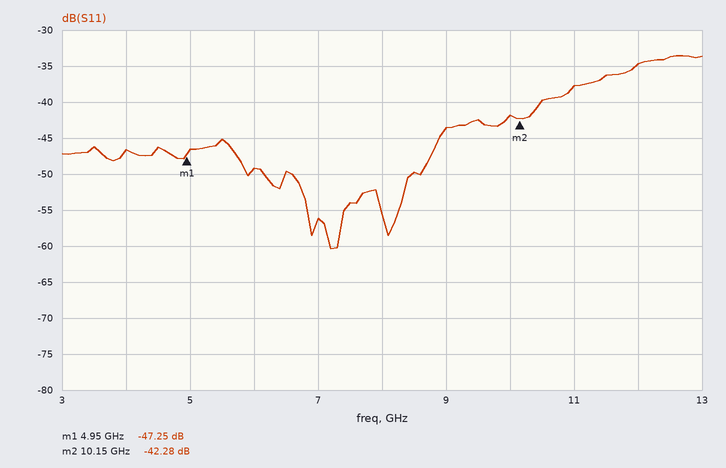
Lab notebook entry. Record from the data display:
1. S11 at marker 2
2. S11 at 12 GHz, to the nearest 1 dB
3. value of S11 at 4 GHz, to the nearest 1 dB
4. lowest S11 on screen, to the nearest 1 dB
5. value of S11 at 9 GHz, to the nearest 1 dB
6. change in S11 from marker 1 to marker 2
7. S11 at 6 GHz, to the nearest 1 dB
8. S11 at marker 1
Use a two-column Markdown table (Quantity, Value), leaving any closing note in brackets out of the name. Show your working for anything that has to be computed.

| Quantity | Value |
|---|---|
| S11 at marker 2 | -42.28 dB |
| S11 at 12 GHz, to the nearest 1 dB | -35 dB |
| value of S11 at 4 GHz, to the nearest 1 dB | -47 dB |
| lowest S11 on screen, to the nearest 1 dB | -60 dB |
| value of S11 at 9 GHz, to the nearest 1 dB | -44 dB |
| change in S11 from marker 1 to marker 2 | -42.28 − (-47.25) = 4.97 dB |
| S11 at 6 GHz, to the nearest 1 dB | -49 dB |
| S11 at marker 1 | -47.25 dB |
